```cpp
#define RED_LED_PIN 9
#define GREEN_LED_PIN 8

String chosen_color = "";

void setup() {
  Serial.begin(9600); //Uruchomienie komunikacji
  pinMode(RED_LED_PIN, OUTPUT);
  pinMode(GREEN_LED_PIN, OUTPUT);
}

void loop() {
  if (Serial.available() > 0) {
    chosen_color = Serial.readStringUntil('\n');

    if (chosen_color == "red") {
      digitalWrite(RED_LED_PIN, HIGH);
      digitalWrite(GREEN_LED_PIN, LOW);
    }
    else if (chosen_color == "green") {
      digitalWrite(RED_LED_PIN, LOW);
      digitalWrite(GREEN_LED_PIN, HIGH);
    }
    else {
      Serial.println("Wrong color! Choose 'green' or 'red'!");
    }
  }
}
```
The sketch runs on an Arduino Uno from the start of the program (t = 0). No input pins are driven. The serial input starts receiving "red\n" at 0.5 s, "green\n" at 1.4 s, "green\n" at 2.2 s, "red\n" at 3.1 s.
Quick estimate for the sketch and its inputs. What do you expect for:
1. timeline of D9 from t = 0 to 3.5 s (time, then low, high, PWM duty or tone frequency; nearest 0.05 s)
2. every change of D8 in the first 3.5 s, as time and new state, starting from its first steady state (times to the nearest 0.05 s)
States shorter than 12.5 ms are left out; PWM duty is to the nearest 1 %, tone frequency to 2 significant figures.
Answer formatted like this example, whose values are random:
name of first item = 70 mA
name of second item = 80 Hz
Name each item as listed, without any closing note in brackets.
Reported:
timeline of D9 from t = 0 to 3.5 s = 0 s low; 0.5 s high; 1.4 s low; 3.1 s high
every change of D8 in the first 3.5 s, as time and new state, starting from its first steady state = 0 s low; 1.4 s high; 3.1 s low
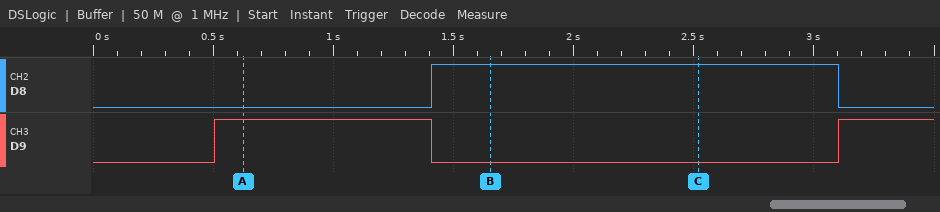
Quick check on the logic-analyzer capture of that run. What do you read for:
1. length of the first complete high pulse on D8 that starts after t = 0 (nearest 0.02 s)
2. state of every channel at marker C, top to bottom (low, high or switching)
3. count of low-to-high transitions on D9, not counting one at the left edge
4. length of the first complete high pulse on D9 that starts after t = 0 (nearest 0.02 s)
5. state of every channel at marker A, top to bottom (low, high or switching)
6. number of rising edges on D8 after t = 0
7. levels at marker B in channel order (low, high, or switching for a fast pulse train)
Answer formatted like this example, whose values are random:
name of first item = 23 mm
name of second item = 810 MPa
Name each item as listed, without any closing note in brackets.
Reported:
length of the first complete high pulse on D8 that starts after t = 0 = 1.70 s
state of every channel at marker C, top to bottom = D8 high, D9 low
count of low-to-high transitions on D9, not counting one at the left edge = 2
length of the first complete high pulse on D9 that starts after t = 0 = 0.90 s
state of every channel at marker A, top to bottom = D8 low, D9 high
number of rising edges on D8 after t = 0 = 1
levels at marker B in channel order = D8 high, D9 low
